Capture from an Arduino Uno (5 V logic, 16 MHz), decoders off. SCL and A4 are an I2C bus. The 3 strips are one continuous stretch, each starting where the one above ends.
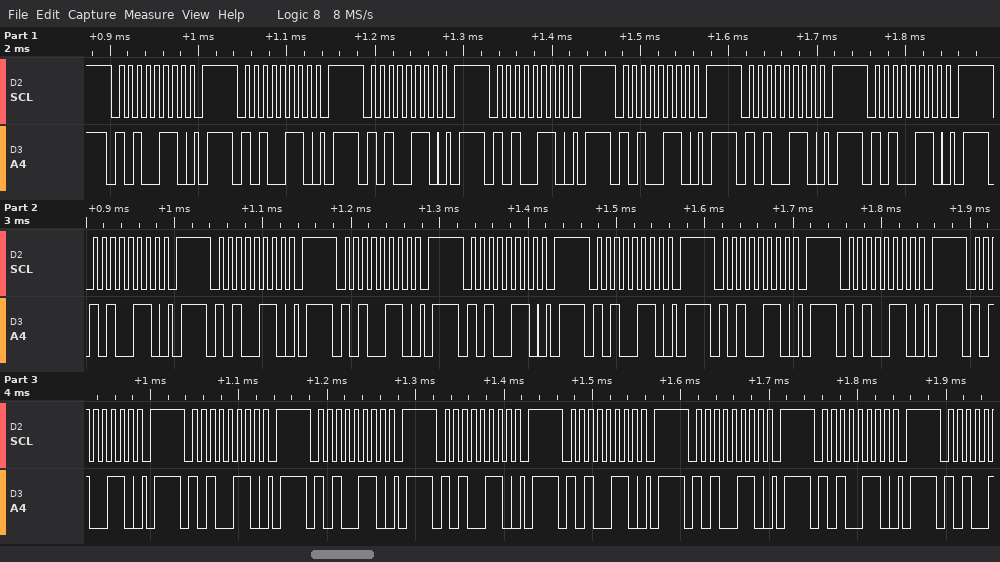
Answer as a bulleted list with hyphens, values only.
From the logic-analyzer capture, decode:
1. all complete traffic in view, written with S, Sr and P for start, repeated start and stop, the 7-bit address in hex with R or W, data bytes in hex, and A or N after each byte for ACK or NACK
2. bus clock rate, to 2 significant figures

- S 53W A P S 53W A P S 53W A P S 53W A P S 53W A P S 53W A P S 53W A P S 53W A P S 53W A P S 53W A P S 53W A P S 53W A P S 53W A P S 53W A P S 53W A P S 53W A P S 53W A P S 53W A P S 53W A P S 53W A P S 53W A P
- 100 kHz
